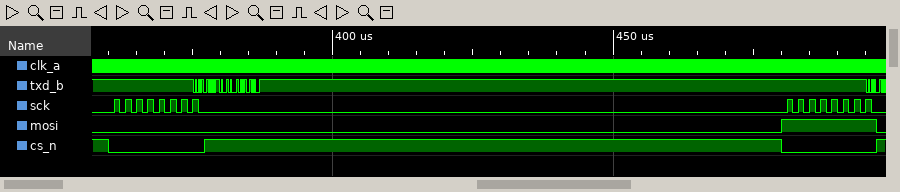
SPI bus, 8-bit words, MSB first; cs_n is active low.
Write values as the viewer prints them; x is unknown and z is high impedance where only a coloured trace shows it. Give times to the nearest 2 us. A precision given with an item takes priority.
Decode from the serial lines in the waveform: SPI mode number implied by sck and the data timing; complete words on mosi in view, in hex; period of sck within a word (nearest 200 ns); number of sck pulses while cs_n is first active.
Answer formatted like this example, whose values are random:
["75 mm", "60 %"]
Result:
["0", "00, FF", "2000 ns", "8"]
